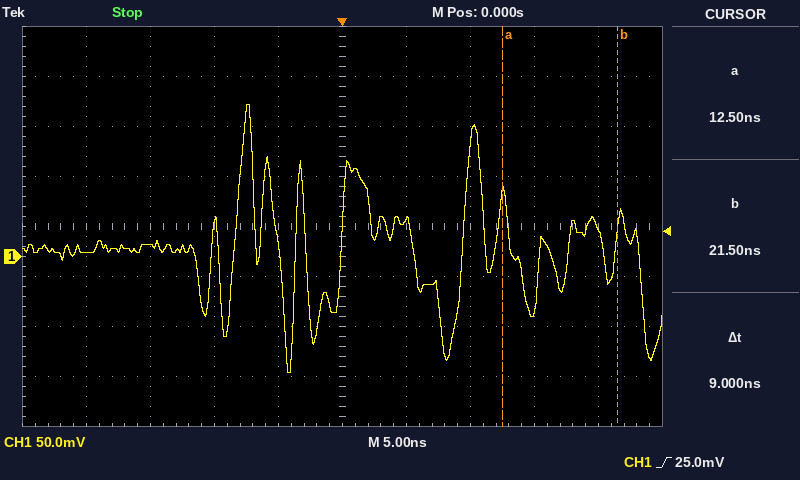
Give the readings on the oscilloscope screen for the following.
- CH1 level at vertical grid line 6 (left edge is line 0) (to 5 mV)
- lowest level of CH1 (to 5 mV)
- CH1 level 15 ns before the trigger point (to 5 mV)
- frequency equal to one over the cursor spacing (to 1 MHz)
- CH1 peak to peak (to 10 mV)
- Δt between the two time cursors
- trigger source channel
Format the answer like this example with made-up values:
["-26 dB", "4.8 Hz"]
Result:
["35 mV", "-115 mV", "10 mV", "111 MHz", "270 mV", "9 ns", "CH1"]
